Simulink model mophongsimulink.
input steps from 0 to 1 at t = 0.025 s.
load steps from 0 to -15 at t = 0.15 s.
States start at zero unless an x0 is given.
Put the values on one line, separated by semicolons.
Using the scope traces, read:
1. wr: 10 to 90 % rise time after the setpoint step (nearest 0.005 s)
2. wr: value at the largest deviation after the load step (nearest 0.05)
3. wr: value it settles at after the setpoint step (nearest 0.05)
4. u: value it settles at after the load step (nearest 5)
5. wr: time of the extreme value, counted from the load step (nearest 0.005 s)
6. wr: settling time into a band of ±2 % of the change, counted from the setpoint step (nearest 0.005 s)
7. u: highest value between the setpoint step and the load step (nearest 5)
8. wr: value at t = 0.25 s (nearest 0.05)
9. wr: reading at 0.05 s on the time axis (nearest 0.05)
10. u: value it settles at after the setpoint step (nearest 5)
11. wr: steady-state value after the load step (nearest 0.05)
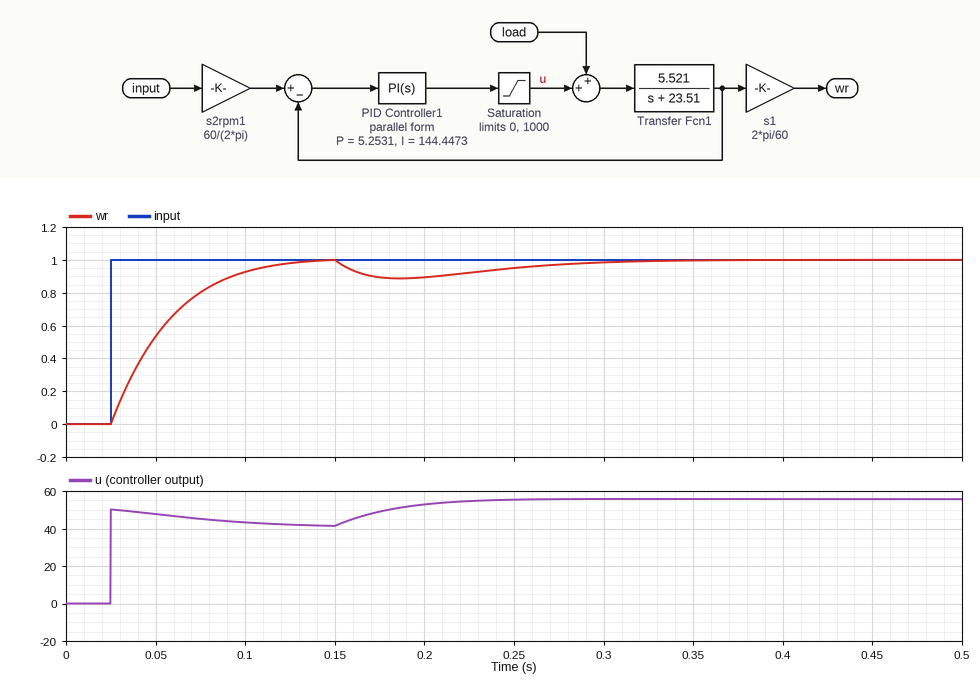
0.065 s; 0.90; 1.00; 55; 0.035 s; 0.100 s; 50; 0.95; 0.55; 40; 1.00
